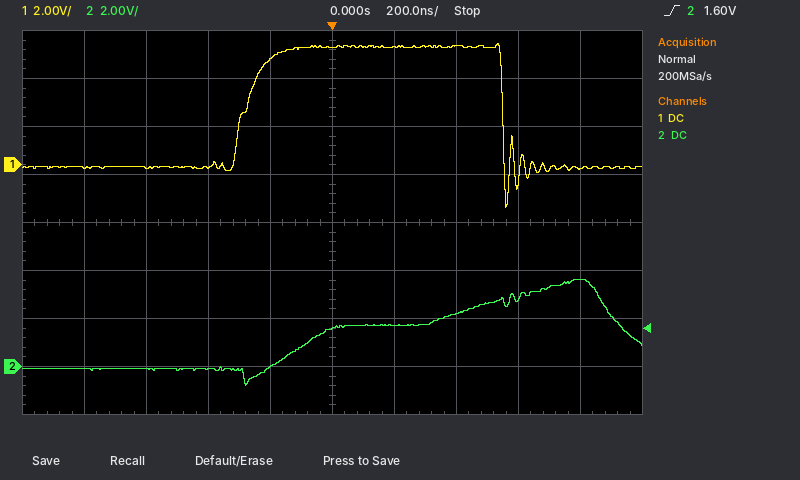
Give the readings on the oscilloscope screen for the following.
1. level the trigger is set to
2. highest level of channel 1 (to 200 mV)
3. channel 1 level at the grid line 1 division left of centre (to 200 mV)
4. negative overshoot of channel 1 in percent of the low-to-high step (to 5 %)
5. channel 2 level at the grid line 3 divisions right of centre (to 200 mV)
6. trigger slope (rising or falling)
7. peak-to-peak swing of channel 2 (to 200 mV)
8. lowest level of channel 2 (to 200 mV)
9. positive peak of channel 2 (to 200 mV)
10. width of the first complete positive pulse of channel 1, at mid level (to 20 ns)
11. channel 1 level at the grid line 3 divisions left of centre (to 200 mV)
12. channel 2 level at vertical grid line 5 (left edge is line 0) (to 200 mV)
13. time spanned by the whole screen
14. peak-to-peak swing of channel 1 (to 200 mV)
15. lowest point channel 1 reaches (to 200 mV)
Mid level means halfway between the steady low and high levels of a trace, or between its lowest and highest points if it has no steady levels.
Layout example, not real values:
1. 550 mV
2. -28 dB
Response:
1. 1.60 V
2. 5.0 V
3. 4.4 V
4. 35 %
5. 2.8 V
6. rising
7. 4.4 V
8. -800 mV
9. 3.6 V
10. 820 ns
11. -200 mV
12. 1.6 V
13. 2 µs
14. 6.8 V
15. -1.8 V
